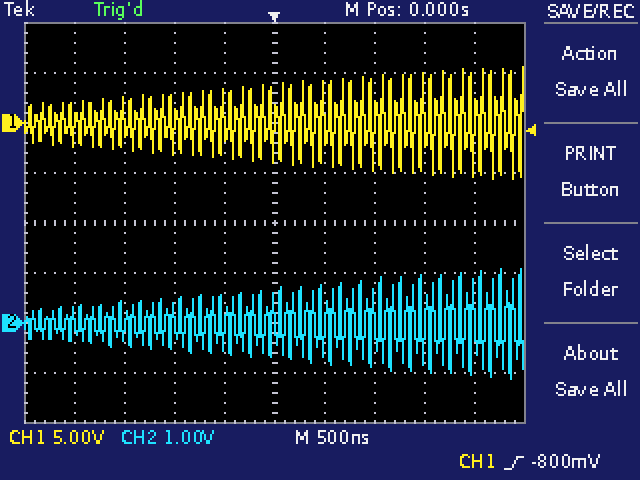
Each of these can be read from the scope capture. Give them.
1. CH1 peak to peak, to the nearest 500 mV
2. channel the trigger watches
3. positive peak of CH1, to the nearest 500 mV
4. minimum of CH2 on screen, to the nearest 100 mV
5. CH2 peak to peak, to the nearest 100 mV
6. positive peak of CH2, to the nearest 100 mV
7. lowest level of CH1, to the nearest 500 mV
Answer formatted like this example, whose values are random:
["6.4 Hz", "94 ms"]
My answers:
["11.0 V", "CH1", "5.5 V", "-1.1 V", "2.2 V", "1.1 V", "-5.5 V"]
